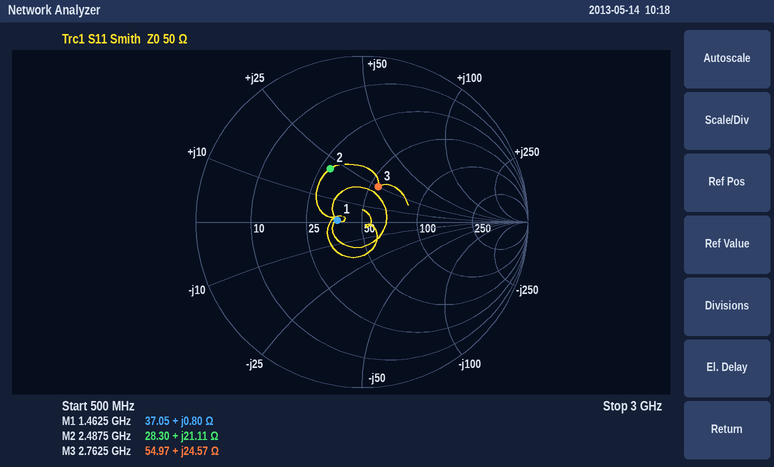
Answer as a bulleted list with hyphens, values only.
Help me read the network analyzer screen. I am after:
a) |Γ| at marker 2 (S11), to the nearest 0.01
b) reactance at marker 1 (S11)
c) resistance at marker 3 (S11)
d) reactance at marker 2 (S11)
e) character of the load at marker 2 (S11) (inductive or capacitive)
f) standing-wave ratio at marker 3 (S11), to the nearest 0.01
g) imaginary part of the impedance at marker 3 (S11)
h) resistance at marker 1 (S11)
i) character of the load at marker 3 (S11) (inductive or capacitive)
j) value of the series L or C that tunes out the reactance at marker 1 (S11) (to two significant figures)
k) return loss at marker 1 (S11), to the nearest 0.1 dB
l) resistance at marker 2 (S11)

- 0.37
- +0.80 Ω
- 54.97 Ω
- +21.11 Ω
- inductive
- 1.61
- +24.57 Ω
- 37.05 Ω
- inductive
- 140 pF
- 16.5 dB
- 28.30 Ω
